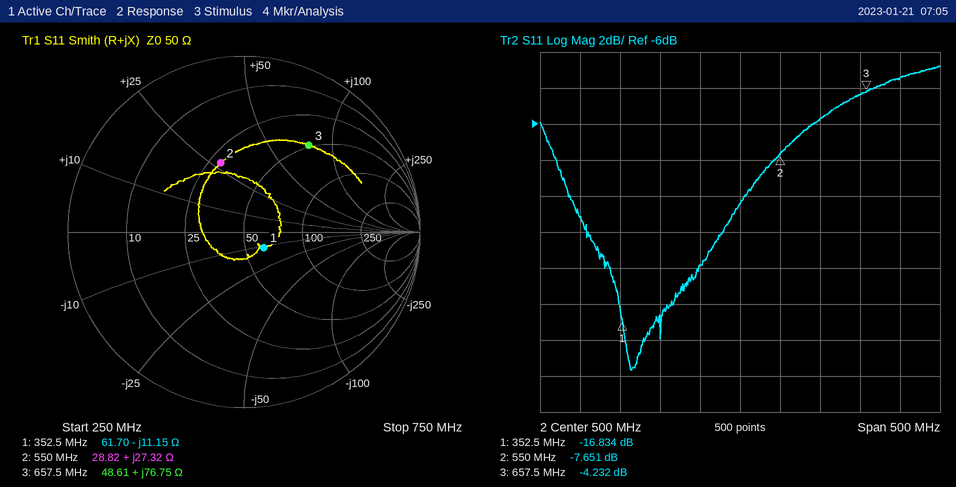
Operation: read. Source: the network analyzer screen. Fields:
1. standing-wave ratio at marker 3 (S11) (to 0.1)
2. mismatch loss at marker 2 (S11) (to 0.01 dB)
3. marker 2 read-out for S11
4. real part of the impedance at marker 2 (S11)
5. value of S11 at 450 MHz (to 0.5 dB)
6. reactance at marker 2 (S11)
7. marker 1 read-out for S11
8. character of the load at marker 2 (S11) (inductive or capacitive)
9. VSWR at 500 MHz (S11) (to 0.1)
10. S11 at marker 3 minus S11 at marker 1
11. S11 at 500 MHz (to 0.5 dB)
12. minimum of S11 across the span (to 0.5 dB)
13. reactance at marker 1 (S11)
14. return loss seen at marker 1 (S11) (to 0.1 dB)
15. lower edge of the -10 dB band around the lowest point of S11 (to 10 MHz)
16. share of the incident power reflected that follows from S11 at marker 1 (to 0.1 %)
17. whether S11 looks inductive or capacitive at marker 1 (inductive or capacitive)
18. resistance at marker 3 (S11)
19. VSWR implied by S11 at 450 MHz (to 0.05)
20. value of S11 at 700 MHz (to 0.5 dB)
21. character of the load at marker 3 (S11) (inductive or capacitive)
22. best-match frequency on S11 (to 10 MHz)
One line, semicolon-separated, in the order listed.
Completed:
4.2; 0.82 dB; -7.651 dB; 28.82 Ω; -14.0 dB; +27.32 Ω; -16.834 dB; inductive; 1.9; 12.602 dB; -10.5 dB; -19.5 dB; -11.15 Ω; 16.8 dB; 290 MHz; 2.1 %; capacitive; 48.61 Ω; 1.50; -3.5 dB; inductive; 360 MHz
